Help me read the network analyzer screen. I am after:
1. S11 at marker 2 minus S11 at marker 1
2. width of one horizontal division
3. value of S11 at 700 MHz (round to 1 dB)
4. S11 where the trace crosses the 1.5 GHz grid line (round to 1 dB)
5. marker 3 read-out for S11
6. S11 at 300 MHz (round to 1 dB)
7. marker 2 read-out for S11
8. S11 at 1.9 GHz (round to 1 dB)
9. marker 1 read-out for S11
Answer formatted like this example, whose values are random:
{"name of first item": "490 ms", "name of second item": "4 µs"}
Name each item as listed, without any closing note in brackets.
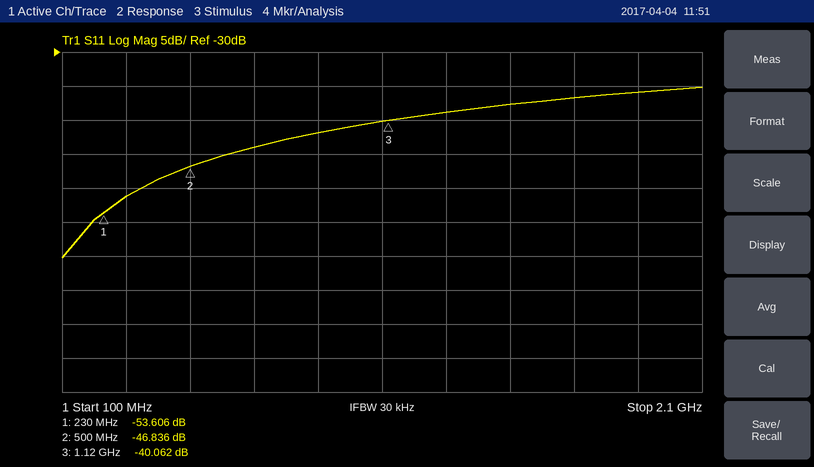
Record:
{"S11 at marker 2 minus S11 at marker 1": "6.770 dB", "width of one horizontal division": "200 MHz", "value of S11 at 700 MHz": "-44 dB", "S11 where the trace crosses the 1.5 GHz grid line": "-38 dB", "marker 3 read-out for S11": "-40.062 dB", "S11 at 300 MHz": "-51 dB", "marker 2 read-out for S11": "-46.836 dB", "S11 at 1.9 GHz": "-36 dB", "marker 1 read-out for S11": "-53.606 dB"}
